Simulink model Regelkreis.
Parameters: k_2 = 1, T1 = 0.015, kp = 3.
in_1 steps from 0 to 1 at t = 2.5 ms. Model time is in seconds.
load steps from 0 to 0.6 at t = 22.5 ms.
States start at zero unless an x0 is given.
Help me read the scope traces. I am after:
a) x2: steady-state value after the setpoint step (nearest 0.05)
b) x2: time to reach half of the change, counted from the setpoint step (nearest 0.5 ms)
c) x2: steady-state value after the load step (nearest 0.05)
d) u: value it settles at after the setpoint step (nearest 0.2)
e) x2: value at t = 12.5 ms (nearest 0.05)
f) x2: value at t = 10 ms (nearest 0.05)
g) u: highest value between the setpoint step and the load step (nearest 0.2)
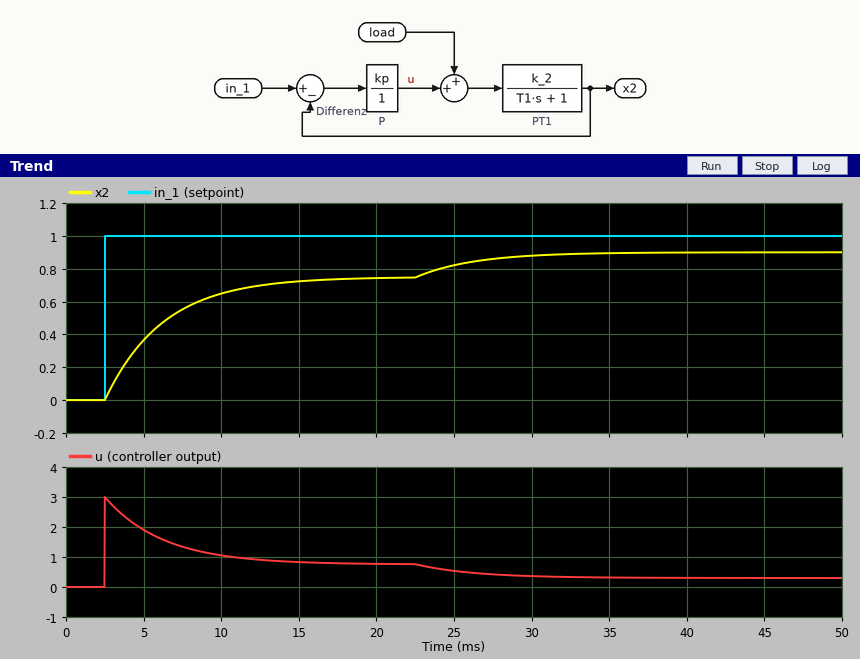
0.75
2.5 ms
0.90
0.8
0.70
0.65
3.0
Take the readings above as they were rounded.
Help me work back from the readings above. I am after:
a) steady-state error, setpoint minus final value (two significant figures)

0.25
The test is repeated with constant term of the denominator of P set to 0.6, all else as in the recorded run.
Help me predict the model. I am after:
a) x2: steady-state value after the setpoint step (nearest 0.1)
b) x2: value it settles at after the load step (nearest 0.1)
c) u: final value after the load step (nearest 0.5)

0.8
0.9
0.5
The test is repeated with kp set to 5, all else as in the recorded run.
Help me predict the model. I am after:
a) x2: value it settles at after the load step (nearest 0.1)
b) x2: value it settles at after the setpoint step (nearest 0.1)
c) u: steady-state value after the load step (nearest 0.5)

0.9
0.8
0.5
